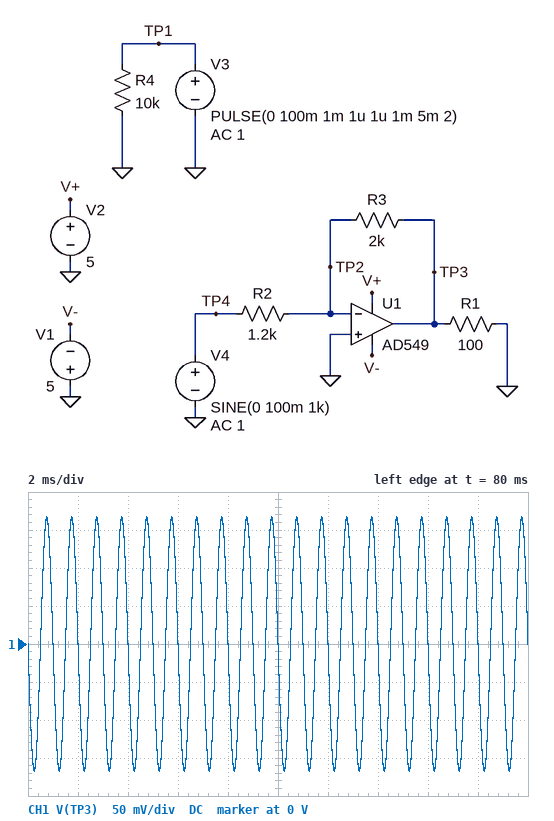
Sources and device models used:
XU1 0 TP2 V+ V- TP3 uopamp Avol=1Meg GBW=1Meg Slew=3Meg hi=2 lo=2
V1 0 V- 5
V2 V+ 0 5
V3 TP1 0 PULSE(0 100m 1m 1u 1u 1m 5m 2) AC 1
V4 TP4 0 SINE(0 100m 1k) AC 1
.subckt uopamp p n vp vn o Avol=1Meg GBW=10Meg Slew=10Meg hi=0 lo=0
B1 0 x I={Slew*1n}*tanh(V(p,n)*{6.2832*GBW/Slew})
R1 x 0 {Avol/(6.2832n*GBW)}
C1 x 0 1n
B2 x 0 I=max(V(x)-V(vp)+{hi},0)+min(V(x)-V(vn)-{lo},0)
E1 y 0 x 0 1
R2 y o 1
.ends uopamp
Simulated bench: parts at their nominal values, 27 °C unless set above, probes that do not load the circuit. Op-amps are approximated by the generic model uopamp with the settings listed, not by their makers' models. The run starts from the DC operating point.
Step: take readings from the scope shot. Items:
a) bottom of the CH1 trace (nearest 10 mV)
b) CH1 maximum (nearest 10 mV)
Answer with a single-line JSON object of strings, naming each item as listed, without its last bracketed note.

{"bottom of the CH1 trace": "-170 mV", "CH1 maximum": "170 mV"}
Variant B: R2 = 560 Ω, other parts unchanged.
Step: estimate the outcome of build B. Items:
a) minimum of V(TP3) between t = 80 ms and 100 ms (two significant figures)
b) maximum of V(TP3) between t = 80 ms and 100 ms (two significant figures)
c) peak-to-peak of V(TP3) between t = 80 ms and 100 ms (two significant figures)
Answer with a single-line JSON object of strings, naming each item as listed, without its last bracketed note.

{"minimum of V(TP3) between t = 80 ms and 100 ms": "-360 mV", "maximum of V(TP3) between t = 80 ms and 100 ms": "360 mV", "peak-to-peak of V(TP3) between t = 80 ms and 100 ms": "710 mV"}
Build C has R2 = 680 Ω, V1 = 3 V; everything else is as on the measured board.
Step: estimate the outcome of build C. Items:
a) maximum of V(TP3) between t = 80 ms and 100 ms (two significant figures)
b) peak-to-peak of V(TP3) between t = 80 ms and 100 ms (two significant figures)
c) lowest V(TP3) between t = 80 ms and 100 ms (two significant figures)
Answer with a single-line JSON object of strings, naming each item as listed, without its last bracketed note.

{"maximum of V(TP3) between t = 80 ms and 100 ms": "290 mV", "peak-to-peak of V(TP3) between t = 80 ms and 100 ms": "590 mV", "lowest V(TP3) between t = 80 ms and 100 ms": "-290 mV"}
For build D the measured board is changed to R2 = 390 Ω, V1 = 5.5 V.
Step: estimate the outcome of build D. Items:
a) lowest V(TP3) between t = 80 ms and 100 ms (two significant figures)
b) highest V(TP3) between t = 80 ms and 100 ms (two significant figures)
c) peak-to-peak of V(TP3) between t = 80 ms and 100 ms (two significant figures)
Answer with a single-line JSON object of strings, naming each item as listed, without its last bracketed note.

{"lowest V(TP3) between t = 80 ms and 100 ms": "-510 mV", "highest V(TP3) between t = 80 ms and 100 ms": "510 mV", "peak-to-peak of V(TP3) between t = 80 ms and 100 ms": "1.0 V"}
